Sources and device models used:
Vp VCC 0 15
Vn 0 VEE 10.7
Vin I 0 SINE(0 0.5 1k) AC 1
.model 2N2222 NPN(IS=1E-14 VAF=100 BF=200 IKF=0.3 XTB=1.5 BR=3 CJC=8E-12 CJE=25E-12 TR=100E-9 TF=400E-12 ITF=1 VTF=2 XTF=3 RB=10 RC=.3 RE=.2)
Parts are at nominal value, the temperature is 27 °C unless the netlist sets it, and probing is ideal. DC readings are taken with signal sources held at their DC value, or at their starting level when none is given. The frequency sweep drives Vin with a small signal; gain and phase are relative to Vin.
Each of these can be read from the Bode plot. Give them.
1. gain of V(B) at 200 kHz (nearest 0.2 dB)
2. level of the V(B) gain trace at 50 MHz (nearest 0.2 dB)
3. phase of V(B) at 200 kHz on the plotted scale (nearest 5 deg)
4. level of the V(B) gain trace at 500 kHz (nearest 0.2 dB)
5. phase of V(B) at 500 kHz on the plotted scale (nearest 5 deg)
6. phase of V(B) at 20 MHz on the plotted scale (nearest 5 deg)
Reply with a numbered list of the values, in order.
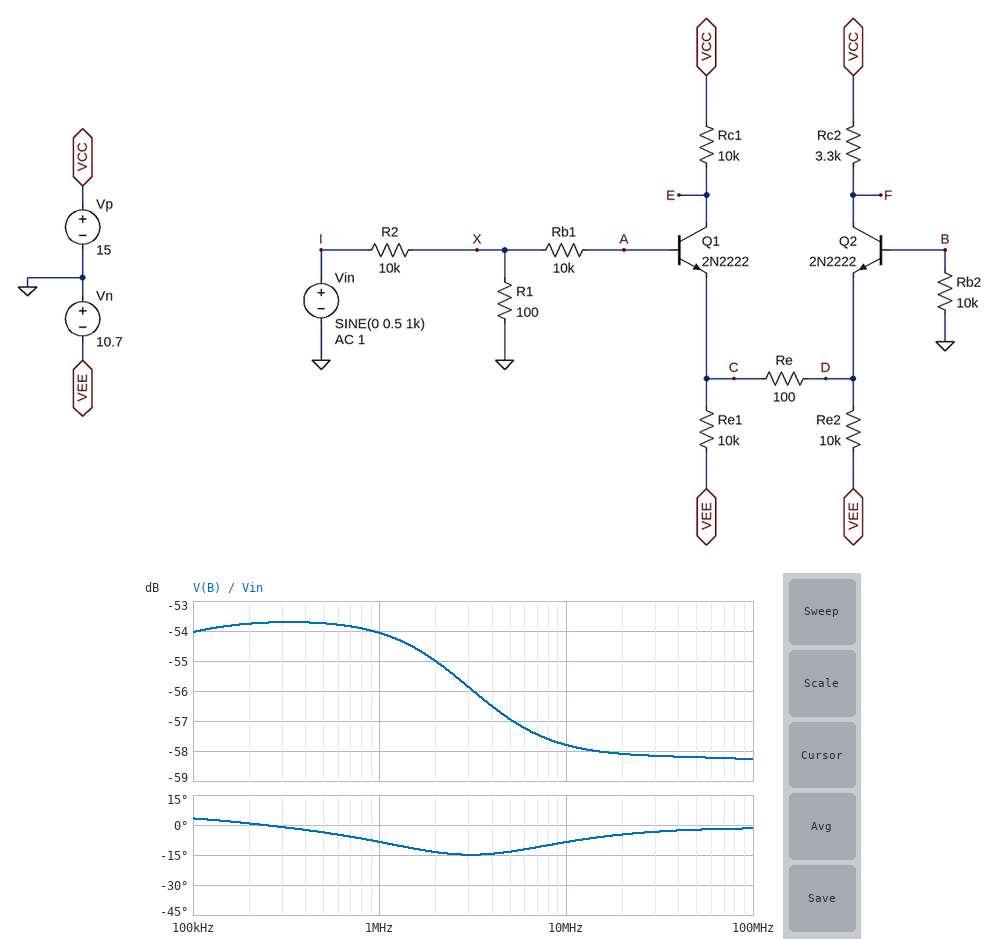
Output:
1. -53.8 dB
2. -58.2 dB
3. 0 deg
4. -53.8 dB
5. -5 deg
6. -5 deg
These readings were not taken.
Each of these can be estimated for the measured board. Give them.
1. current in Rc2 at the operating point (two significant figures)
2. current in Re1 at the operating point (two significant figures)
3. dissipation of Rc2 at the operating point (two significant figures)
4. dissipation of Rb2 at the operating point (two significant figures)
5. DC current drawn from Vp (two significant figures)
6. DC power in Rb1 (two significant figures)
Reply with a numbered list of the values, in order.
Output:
1. 1.0 mA
2. 1.0 mA
3. 3.4 mW
4. 210 nW
5. 2.0 mA
6. 220 nW
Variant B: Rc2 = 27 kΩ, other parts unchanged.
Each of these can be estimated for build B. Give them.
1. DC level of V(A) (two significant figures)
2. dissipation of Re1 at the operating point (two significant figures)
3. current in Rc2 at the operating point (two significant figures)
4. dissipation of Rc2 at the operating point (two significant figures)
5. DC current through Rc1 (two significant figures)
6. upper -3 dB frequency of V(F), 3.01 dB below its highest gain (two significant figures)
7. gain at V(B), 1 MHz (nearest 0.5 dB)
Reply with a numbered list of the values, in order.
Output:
1. -70 mV
2. 9.9 mW
3. 580 µA
4. 9.1 mW
5. 1.4 mA
6. 430 kHz
7. -47.0 dB
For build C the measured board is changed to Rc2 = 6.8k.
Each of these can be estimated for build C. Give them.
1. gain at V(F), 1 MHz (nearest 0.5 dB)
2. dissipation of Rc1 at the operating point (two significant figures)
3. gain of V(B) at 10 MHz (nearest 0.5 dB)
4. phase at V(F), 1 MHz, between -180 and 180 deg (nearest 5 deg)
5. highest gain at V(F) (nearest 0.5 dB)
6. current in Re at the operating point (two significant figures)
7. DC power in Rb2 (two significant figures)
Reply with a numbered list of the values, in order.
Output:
1. -37.5 dB
2. 9.7 mW
3. -56.0 dB
4. -90 deg
5. -12.0 dB
6. 10 µA
7. 220 nW
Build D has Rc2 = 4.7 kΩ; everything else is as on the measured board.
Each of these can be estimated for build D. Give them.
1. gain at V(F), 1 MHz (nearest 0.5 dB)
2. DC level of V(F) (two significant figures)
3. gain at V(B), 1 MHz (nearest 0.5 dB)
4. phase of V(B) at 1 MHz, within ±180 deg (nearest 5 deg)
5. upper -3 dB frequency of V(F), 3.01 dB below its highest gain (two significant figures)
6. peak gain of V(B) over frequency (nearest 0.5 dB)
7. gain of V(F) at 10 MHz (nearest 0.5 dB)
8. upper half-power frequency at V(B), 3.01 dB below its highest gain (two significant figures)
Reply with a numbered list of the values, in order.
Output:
1. -39.0 dB
2. 10 V
3. -52.0 dB
4. -10 deg
5. 67 kHz
6. -51.5 dB
7. -57.0 dB
8. 2.9 MHz
